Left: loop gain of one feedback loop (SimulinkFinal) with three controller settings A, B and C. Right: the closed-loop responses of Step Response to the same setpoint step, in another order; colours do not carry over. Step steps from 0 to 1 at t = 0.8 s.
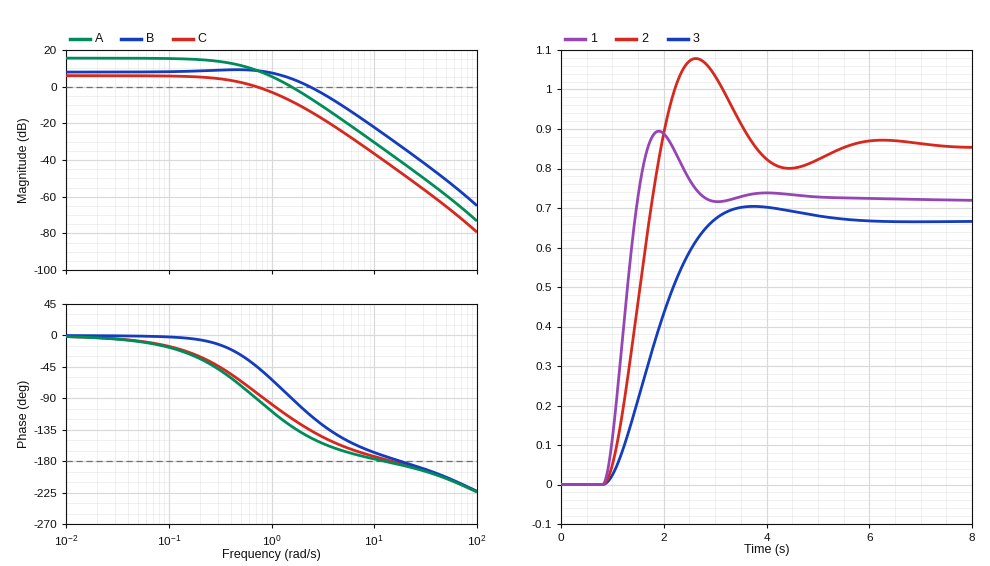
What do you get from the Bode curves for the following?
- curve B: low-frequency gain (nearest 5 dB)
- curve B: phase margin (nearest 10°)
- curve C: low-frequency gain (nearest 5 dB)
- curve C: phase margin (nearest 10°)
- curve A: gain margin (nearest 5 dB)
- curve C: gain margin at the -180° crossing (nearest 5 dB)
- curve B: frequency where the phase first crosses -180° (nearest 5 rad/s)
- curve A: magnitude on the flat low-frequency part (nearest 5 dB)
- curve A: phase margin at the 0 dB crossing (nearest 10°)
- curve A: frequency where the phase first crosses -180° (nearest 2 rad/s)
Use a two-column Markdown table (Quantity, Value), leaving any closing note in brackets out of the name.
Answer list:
| Quantity | Value |
|---|---|
| curve B: low-frequency gain | 10 dB |
| curve B: phase margin | 70° |
| curve C: low-frequency gain | 5 dB |
| curve C: phase margin | 100° |
| curve A: gain margin | 35 dB |
| curve C: gain margin at the -180° crossing | 45 dB |
| curve B: frequency where the phase first crosses -180° | 20 rad/s |
| curve A: magnitude on the flat low-frequency part | 15 dB |
| curve A: phase margin at the 0 dB crossing | 50° |
| curve A: frequency where the phase first crosses -180° | 12 rad/s |
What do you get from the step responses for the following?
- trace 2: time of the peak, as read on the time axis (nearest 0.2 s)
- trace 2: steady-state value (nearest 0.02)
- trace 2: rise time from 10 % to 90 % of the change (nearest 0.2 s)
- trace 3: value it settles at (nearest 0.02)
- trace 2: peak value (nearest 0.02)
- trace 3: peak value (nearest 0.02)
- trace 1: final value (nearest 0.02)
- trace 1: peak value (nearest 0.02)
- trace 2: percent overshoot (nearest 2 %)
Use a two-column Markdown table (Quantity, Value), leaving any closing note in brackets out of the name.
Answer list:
| Quantity | Value |
|---|---|
| trace 2: time of the peak, as read on the time axis | 2.6 s |
| trace 2: steady-state value | 0.86 |
| trace 2: rise time from 10 % to 90 % of the change | 0.8 s |
| trace 3: value it settles at | 0.66 |
| trace 2: peak value | 1.08 |
| trace 3: peak value | 0.70 |
| trace 1: final value | 0.72 |
| trace 1: peak value | 0.90 |
| trace 2: percent overshoot | 26 % |
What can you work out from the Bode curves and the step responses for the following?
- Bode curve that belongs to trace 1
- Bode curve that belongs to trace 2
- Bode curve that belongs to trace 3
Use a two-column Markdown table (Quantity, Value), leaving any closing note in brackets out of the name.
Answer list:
| Quantity | Value |
|---|---|
| Bode curve that belongs to trace 1 | B |
| Bode curve that belongs to trace 2 | A |
| Bode curve that belongs to trace 3 | C |
